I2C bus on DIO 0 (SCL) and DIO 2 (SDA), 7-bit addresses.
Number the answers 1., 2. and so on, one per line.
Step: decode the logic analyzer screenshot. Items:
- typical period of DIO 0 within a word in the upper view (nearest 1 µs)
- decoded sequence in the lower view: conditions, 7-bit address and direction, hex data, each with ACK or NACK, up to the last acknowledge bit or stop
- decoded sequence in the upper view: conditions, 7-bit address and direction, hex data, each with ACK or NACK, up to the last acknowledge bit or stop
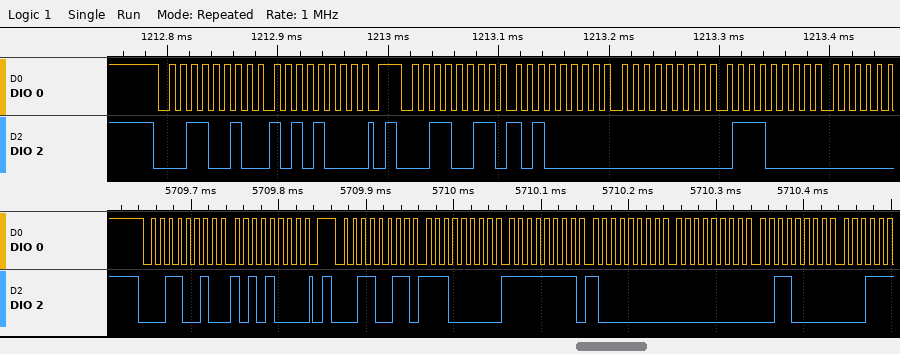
1. 10 µs
2. start, address 19 write ACK, A8 ACK, stop, start, address 19 read ACK, E0 ACK, FF ACK, 80 ACK, 00 ACK, 30 ACK
3. start, address 19 write ACK, A8 ACK, stop, start, address 19 read ACK, A0 ACK, 00 ACK, 70 ACK
